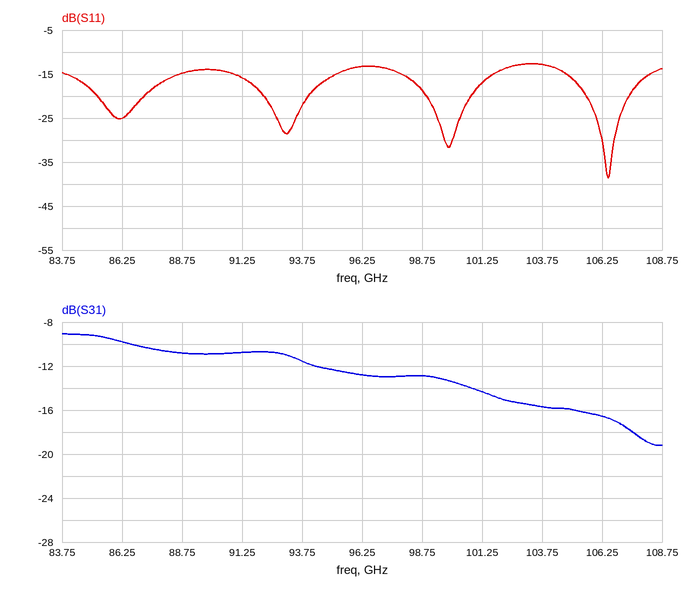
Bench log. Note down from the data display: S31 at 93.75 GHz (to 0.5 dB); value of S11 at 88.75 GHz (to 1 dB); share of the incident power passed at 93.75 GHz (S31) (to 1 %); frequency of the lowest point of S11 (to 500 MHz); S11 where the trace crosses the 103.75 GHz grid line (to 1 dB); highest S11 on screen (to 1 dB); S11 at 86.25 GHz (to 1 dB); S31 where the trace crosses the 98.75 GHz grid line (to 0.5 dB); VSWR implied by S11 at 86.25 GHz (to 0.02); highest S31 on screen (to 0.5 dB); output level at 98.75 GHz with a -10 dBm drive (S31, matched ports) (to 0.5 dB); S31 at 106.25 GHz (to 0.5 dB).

-11.5 dB
-15 dB
7 %
106.5 GHz
-13 dB
-13 dB
-25 dB
-13.0 dB
1.12
-9.0 dB
-23.0 dBm
-16.5 dB
